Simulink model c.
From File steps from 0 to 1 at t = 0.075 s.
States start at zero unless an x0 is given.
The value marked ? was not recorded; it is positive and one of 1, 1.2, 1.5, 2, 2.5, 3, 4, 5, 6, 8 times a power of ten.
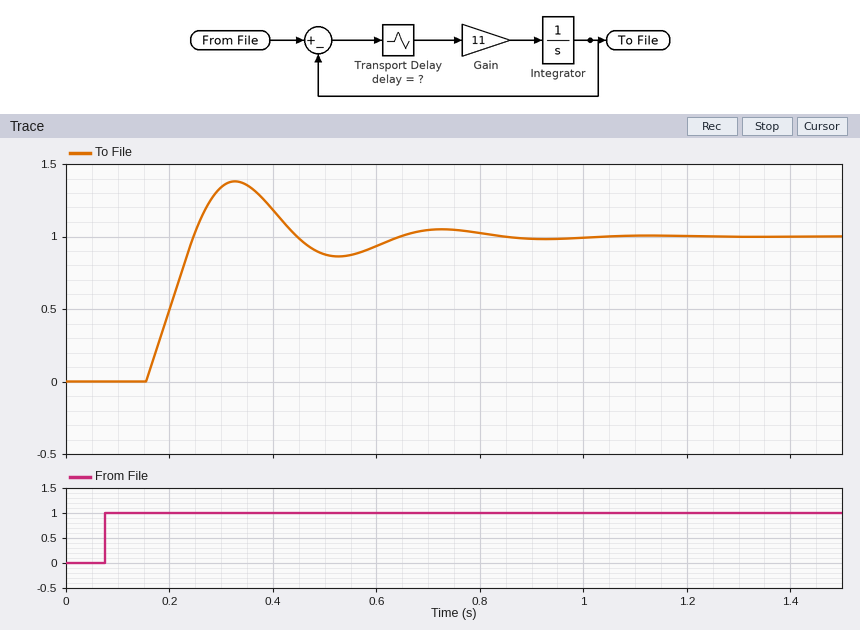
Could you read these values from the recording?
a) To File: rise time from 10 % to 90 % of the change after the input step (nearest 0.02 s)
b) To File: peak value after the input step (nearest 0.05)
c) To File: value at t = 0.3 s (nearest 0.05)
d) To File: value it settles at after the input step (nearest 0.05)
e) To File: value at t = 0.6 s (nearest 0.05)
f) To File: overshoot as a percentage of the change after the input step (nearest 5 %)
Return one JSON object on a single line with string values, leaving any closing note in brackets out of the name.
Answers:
{"To File: rise time from 10 % to 90 % of the change after the input step": "0.08 s", "To File: peak value after the input step": "1.40", "To File: value at t = 0.3 s": "1.35", "To File: value it settles at after the input step": "1.00", "To File: value at t = 0.6 s": "0.95", "To File: overshoot as a percentage of the change after the input step": "40 %"}
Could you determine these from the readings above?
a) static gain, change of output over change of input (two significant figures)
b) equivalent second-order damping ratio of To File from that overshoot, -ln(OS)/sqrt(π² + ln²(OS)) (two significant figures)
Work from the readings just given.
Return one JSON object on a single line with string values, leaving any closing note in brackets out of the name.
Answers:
{"static gain, change of output over change of input": "1.0", "equivalent second-order damping ratio of To File from that overshoot, -ln(OS)/sqrt(π² + ln²(OS))": "0.28"}
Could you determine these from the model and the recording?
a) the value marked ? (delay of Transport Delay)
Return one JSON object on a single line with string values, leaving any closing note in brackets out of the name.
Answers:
{"the value marked ?": "0.08"}
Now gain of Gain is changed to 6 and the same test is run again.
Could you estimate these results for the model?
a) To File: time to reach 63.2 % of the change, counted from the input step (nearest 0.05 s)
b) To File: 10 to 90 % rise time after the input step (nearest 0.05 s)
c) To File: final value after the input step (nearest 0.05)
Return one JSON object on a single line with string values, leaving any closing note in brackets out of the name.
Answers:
{"To File: time to reach 63.2 % of the change, counted from the input step": "0.20 s", "To File: 10 to 90 % rise time after the input step": "0.15 s", "To File: final value after the input step": "1.00"}
